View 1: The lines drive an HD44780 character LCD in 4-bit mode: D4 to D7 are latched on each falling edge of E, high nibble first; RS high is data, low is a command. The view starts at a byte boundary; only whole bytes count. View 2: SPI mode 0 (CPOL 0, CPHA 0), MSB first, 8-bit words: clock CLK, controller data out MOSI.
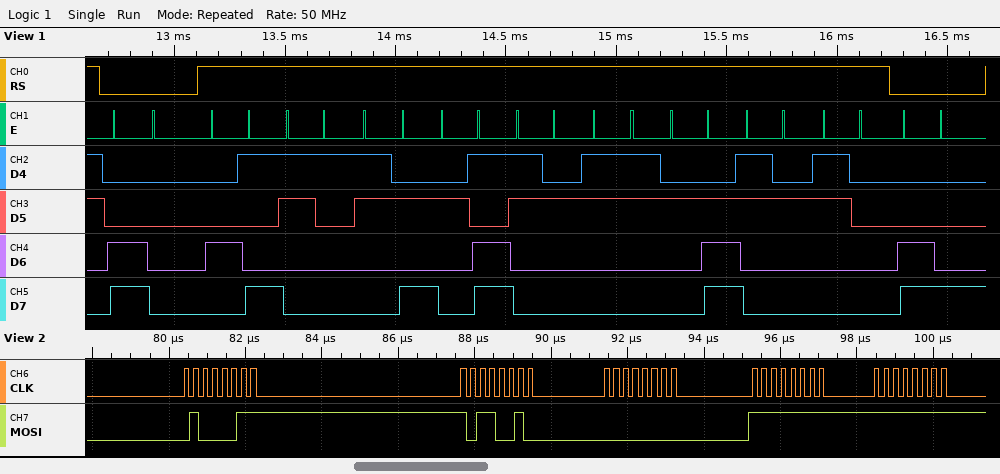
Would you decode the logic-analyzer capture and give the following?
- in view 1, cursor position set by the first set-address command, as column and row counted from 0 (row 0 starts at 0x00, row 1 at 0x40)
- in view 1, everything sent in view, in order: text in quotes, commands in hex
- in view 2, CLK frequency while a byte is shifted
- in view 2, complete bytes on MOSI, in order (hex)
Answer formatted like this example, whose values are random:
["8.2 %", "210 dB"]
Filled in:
["column 0, row 1", "0xC0 \"I1:-23.20\" 0xC8", "4 MHz", "43 B2 00 FF FF"]
